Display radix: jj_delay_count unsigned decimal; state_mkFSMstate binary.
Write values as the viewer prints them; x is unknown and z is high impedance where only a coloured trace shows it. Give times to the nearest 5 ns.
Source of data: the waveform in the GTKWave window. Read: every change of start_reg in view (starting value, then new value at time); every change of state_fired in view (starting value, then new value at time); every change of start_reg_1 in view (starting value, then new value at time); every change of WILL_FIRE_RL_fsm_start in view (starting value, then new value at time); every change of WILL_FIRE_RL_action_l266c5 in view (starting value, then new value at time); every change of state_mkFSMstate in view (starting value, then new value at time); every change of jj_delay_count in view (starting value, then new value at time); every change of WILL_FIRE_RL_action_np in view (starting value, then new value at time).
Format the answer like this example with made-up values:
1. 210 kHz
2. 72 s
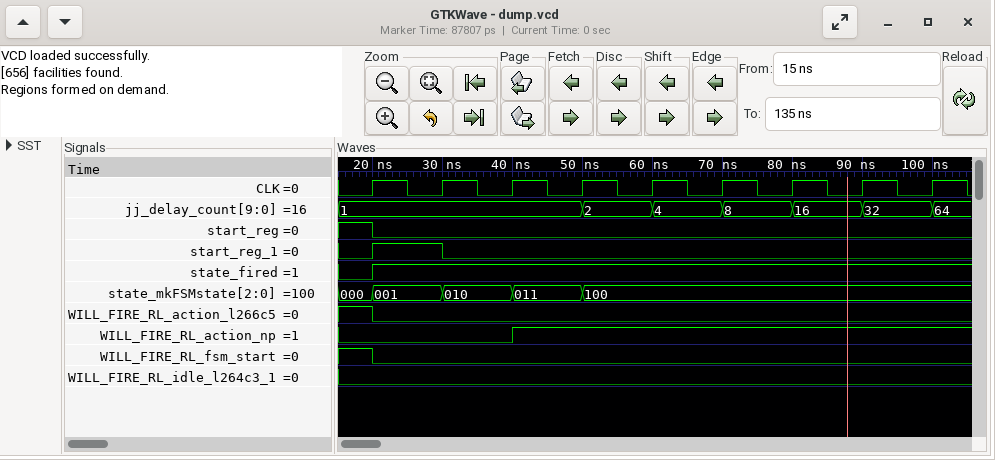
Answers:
1. 1, 0 at 20 ns
2. 0, 1 at 20 ns
3. 0, 1 at 20 ns, 0 at 30 ns
4. 1, 0 at 20 ns
5. 1, 0 at 20 ns
6. 000, 001 at 20 ns, 010 at 30 ns, 011 at 40 ns, 100 at 50 ns
7. 1, 2 at 50 ns, 4 at 60 ns, 8 at 70 ns, 16 at 80 ns, 32 at 90 ns, 64 at 100 ns
8. 0, 1 at 40 ns
